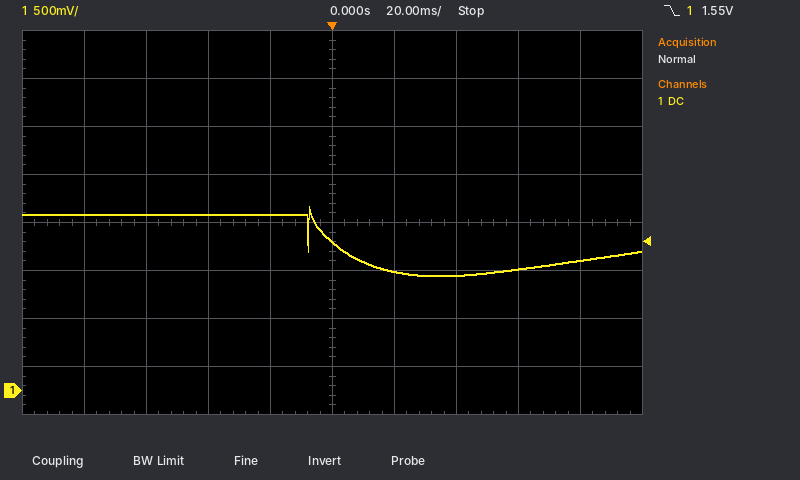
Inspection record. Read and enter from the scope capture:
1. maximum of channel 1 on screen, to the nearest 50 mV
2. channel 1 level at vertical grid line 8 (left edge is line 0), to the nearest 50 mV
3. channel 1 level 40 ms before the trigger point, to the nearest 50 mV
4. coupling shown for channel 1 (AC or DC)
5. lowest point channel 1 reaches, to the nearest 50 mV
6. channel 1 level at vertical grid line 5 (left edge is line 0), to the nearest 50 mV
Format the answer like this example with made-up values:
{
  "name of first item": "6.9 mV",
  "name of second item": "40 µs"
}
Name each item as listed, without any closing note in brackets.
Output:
{
  "maximum of channel 1 on screen, to the nearest 50 mV": "1.90 V",
  "channel 1 level at vertical grid line 8 (left edge is line 0), to the nearest 50 mV": "1.25 V",
  "channel 1 level 40 ms before the trigger point, to the nearest 50 mV": "1.85 V",
  "coupling shown for channel 1": "DC",
  "lowest point channel 1 reaches, to the nearest 50 mV": "1.20 V",
  "channel 1 level at vertical grid line 5 (left edge is line 0), to the nearest 50 mV": "1.55 V"
}
